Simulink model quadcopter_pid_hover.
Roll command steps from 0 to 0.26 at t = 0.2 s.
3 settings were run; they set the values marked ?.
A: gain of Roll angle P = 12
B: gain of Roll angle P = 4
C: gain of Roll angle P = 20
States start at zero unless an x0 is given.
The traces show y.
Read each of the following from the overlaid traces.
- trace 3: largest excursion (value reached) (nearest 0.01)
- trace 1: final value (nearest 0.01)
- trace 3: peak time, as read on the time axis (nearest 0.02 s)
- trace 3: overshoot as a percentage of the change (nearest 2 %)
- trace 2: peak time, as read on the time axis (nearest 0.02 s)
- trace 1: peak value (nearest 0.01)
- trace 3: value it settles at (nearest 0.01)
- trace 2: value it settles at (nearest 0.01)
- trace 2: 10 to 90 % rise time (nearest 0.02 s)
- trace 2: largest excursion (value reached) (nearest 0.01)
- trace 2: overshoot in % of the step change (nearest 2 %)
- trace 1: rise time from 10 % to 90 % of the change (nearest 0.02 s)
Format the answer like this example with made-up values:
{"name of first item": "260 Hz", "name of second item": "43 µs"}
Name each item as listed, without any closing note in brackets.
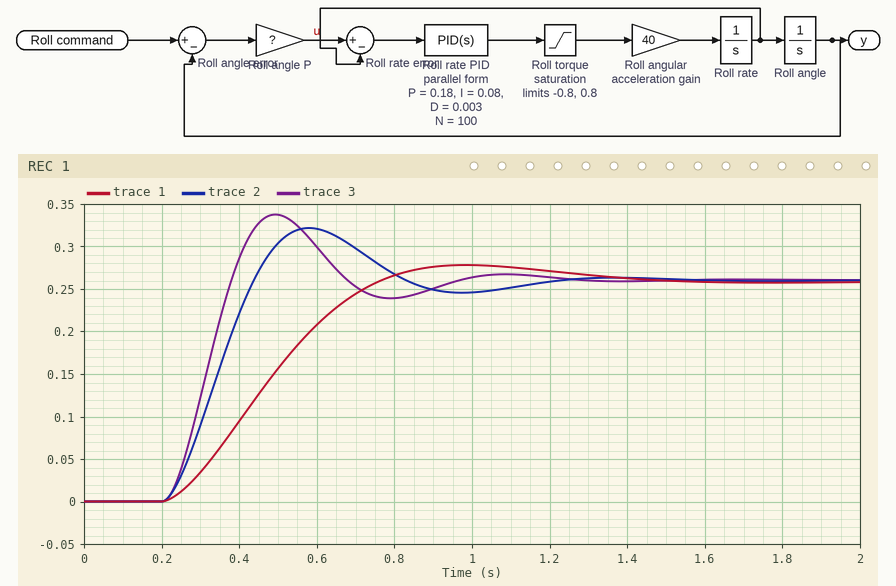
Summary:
{"trace 3: largest excursion (value reached)": "0.34", "trace 1: final value": "0.26", "trace 3: peak time, as read on the time axis": "0.50 s", "trace 3: overshoot as a percentage of the change": "30 %", "trace 2: peak time, as read on the time axis": "0.58 s", "trace 1: peak value": "0.28", "trace 3: value it settles at": "0.26", "trace 2: value it settles at": "0.26", "trace 2: 10 to 90 % rise time": "0.16 s", "trace 2: largest excursion (value reached)": "0.32", "trace 2: overshoot in % of the step change": "24 %", "trace 1: rise time from 10 % to 90 % of the change": "0.38 s"}
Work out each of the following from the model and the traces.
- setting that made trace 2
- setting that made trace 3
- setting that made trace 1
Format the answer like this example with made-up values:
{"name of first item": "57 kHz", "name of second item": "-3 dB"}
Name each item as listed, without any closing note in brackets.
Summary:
{"setting that made trace 2": "A", "setting that made trace 3": "C", "setting that made trace 1": "B"}
